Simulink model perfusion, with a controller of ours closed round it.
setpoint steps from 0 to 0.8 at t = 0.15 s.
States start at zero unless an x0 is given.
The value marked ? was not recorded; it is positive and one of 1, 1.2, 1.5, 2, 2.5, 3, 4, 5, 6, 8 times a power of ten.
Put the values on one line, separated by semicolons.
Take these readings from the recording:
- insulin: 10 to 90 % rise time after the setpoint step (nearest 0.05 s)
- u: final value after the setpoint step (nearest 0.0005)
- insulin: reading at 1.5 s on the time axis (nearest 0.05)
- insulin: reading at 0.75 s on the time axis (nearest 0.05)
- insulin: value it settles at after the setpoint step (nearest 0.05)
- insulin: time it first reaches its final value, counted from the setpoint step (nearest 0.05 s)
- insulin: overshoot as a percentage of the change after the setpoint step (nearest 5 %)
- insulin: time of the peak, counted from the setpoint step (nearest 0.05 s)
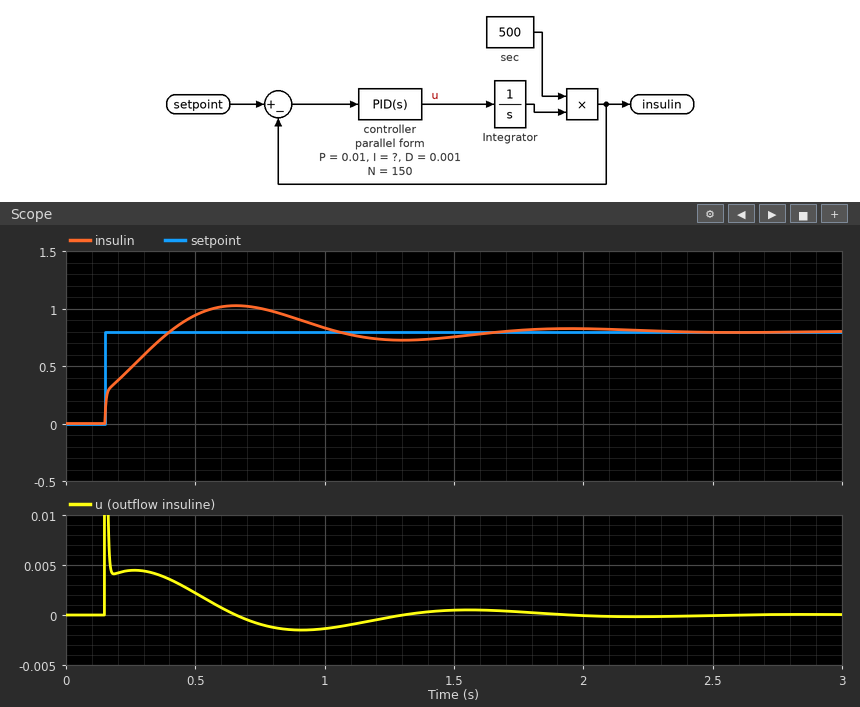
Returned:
0.20 s; 0.0000; 0.75; 1.00; 0.80; 0.25 s; 30 %; 0.50 s
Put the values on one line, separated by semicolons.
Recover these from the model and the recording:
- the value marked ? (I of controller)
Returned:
0.08
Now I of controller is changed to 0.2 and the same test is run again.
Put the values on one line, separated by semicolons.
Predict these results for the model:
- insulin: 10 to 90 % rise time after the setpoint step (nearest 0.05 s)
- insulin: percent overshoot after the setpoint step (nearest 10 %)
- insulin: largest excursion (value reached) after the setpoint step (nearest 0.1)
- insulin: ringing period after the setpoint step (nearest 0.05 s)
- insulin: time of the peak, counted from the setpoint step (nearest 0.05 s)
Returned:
0.15 s; 40 %; 1.1; 0.80 s; 0.35 s
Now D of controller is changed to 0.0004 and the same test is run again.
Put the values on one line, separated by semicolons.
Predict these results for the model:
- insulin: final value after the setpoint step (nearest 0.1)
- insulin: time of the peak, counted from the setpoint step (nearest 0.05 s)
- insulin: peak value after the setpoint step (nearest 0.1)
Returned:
0.8; 0.45 s; 1.1
